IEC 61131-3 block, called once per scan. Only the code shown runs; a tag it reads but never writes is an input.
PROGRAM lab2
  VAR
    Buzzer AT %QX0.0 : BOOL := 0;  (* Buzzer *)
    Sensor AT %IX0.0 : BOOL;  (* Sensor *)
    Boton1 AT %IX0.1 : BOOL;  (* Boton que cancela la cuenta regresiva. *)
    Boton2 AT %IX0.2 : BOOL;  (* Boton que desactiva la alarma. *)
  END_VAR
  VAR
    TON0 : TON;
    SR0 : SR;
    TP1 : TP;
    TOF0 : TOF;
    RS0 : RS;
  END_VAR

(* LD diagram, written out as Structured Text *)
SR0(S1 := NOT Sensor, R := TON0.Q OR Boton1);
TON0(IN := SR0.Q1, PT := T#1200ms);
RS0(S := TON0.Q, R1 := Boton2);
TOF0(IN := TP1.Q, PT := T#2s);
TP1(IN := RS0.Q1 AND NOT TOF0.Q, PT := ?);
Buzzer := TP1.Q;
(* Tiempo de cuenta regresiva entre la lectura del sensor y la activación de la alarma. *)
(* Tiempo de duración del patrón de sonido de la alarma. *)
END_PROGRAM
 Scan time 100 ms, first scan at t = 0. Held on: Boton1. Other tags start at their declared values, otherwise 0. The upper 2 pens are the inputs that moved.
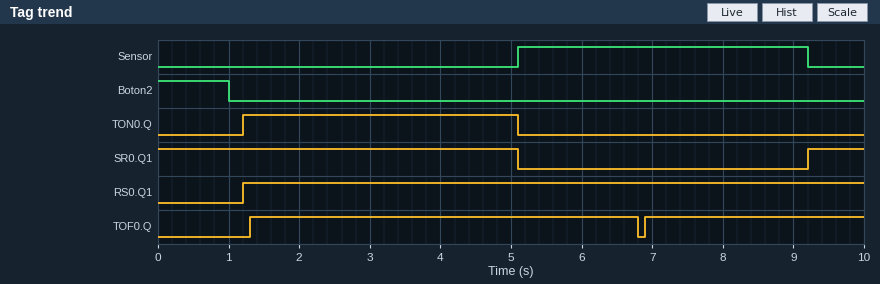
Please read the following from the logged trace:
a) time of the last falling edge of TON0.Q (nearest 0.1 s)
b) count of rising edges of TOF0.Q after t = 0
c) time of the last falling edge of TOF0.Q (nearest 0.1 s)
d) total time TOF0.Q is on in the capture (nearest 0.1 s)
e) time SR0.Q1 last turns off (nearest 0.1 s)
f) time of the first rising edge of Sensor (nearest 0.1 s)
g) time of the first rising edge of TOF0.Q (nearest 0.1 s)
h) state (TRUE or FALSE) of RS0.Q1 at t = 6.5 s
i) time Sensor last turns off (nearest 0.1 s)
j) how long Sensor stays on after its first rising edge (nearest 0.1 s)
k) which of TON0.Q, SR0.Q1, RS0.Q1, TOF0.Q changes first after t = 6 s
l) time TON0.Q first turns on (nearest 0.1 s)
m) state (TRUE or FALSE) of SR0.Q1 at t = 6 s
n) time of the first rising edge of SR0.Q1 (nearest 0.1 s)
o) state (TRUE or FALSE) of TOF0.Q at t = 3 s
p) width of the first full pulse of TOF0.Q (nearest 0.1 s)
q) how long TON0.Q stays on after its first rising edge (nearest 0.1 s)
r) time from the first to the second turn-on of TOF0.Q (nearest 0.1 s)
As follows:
5.1 s
2
6.8 s
8.6 s
5.1 s
5.1 s
1.3 s
TRUE
9.2 s
4.1 s
TOF0.Q
1.2 s
FALSE
9.2 s
TRUE
5.5 s
3.9 s
5.6 s
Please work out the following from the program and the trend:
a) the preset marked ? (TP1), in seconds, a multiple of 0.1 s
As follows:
3.5 s
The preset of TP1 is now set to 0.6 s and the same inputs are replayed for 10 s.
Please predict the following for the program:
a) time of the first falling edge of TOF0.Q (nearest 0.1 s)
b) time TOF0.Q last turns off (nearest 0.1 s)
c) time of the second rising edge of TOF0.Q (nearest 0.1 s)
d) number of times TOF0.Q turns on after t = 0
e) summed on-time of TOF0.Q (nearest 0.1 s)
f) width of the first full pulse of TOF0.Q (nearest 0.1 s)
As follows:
3.9 s
9.3 s
4.0 s
4
8.4 s
2.6 s
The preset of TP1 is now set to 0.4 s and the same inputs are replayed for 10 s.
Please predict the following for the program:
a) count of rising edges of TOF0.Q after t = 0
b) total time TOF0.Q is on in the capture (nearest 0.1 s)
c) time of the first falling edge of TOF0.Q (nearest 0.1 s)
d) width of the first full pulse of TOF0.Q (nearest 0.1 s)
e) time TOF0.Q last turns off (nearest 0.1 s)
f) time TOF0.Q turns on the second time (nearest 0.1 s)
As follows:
4
8.4 s
3.7 s
2.4 s
8.7 s
3.8 s
